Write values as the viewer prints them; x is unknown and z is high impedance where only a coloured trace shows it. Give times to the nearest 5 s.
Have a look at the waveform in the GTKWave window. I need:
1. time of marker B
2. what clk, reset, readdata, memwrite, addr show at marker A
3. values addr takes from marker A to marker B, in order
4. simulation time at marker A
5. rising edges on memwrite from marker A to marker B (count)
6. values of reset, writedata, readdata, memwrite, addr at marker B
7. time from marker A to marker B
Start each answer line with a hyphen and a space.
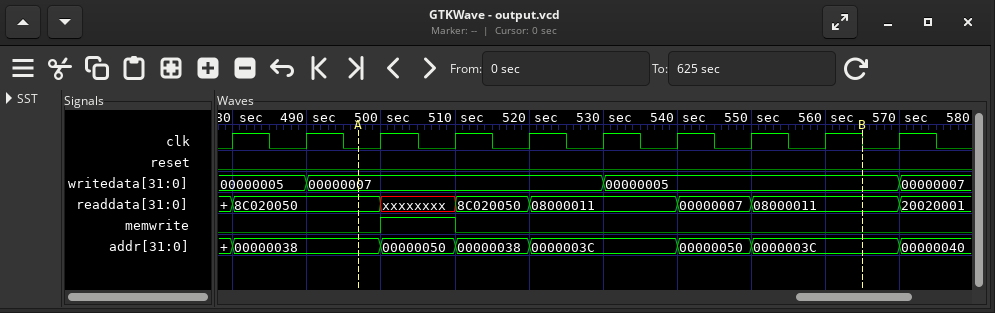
- 565 s
- clk=0, reset=0, readdata=8C020050, memwrite=0, addr=00000038
- 00000038, 00000050, 00000038, 0000003C, 00000050, 0000003C
- 495 s
- 1
- reset=0, writedata=00000005, readdata=08000011, memwrite=0, addr=0000003C
- 70 s
